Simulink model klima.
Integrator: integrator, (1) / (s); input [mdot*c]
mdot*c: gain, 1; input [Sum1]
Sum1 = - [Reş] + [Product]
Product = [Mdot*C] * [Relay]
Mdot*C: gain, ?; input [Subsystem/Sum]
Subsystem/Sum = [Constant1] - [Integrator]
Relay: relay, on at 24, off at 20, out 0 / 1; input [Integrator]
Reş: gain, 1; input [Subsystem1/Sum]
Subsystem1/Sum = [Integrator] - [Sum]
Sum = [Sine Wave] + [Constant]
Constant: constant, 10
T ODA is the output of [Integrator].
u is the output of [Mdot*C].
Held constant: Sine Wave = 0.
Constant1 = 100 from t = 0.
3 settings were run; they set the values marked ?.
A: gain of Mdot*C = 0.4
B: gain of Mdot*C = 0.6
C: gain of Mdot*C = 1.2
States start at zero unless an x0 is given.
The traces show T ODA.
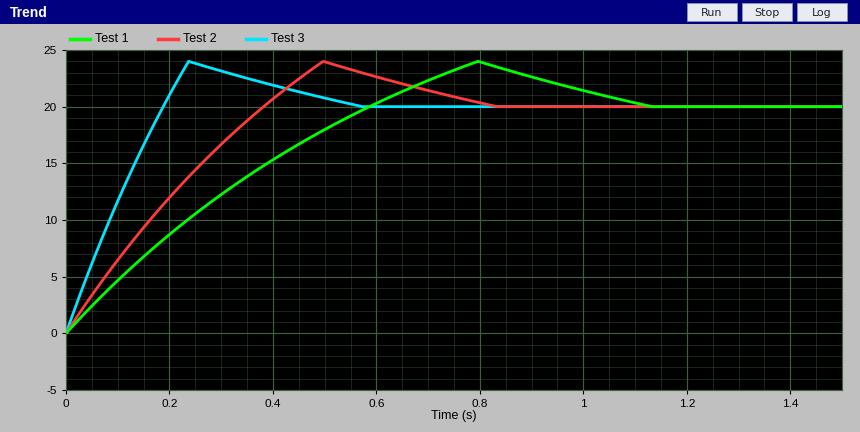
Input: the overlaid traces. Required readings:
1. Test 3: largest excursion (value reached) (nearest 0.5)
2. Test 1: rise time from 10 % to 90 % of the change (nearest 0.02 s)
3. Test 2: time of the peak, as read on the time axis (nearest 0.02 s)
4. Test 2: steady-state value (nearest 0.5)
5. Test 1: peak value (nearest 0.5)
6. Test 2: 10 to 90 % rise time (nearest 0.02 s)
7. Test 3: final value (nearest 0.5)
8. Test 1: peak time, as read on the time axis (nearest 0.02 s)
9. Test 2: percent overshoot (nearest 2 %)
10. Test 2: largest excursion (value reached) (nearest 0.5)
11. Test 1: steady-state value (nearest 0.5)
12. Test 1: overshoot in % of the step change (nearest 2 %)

24.0
0.46 s
0.50 s
20.0
24.0
0.30 s
20.0
0.80 s
20 %
24.0
20.0
20 %
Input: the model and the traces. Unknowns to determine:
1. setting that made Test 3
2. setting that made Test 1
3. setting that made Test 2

C
A
B
